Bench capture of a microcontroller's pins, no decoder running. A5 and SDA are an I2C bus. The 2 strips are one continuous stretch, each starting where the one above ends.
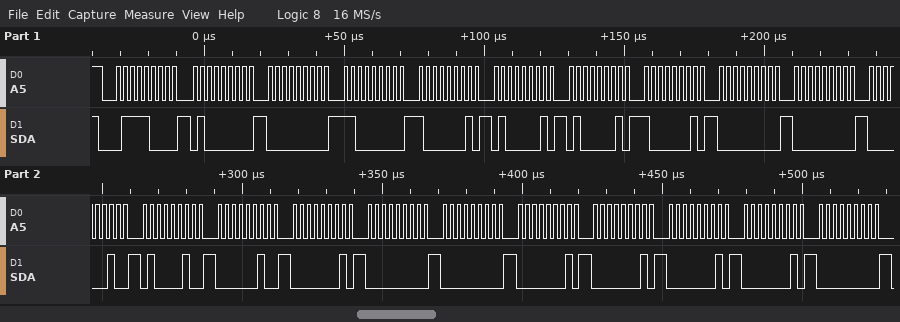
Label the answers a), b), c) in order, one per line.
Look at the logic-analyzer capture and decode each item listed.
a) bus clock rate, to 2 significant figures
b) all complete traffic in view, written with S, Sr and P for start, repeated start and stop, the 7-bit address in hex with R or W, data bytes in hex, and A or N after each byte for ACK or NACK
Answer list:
a) 400 kHz
b) S 3CW A 40 A 00 A C0 A 81 A 41 A 41 A 81 A 00 A 00 A 02 A 42 A 02 A 01 A 00 A 00 A 01 A 01 A 01 A 01 A 00 A
